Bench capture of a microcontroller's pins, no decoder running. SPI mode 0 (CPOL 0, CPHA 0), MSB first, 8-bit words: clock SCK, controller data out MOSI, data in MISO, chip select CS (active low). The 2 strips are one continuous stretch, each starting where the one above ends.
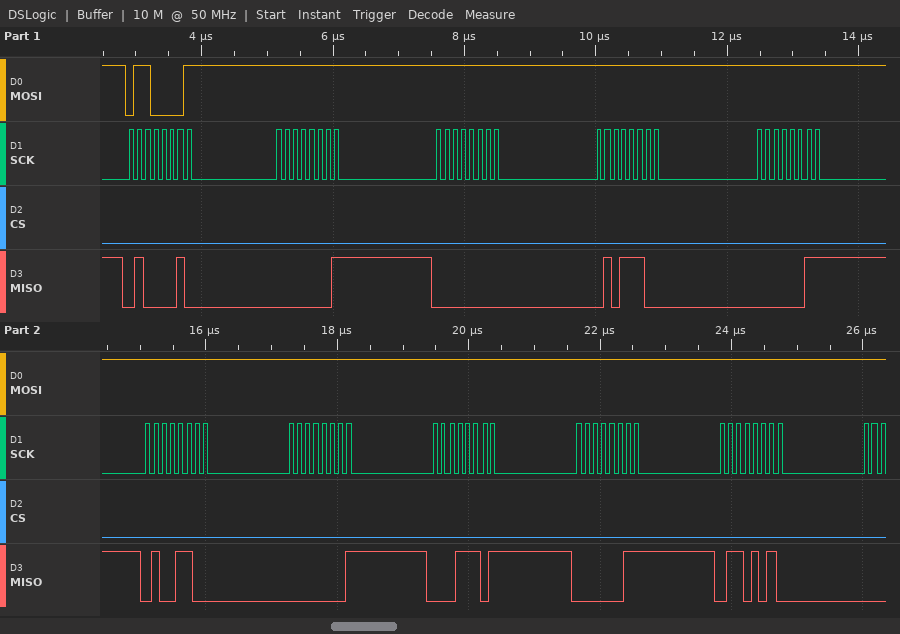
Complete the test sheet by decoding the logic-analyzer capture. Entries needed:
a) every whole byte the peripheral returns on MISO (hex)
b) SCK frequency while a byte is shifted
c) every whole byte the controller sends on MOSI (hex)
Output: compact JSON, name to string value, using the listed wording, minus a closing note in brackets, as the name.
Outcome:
{"every whole byte the peripheral returns on MISO": "0x42 0x01 0x00 0x5C 0x03 0x4C 0x01 0x1D 0x03 0x6A", "SCK frequency while a byte is shifted": "8 MHz", "every whole byte the controller sends on MOSI": "0x61 0xFF 0xFF 0xFF 0xFF 0xFF 0xFF 0xFF 0xFF 0xFF"}
